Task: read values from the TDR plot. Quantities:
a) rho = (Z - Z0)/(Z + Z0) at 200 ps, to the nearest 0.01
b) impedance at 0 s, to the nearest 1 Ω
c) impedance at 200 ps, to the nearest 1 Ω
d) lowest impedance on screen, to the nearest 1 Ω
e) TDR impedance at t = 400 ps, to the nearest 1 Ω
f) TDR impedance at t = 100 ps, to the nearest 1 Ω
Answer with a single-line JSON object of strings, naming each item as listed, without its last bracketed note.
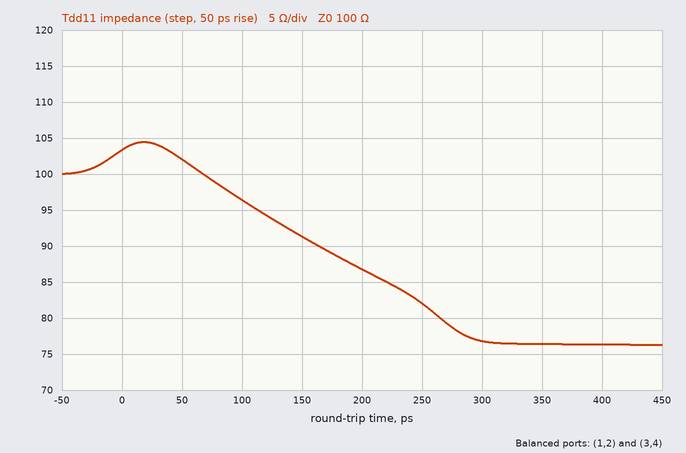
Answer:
{"rho = (Z - Z0)/(Z + Z0) at 200 ps, to the nearest 0.01": "-0.07", "impedance at 0 s, to the nearest 1 Ω": "103 Ω", "impedance at 200 ps, to the nearest 1 Ω": "87 Ω", "lowest impedance on screen, to the nearest 1 Ω": "76 Ω", "TDR impedance at t = 400 ps, to the nearest 1 Ω": "76 Ω", "TDR impedance at t = 100 ps, to the nearest 1 Ω": "96 Ω"}
